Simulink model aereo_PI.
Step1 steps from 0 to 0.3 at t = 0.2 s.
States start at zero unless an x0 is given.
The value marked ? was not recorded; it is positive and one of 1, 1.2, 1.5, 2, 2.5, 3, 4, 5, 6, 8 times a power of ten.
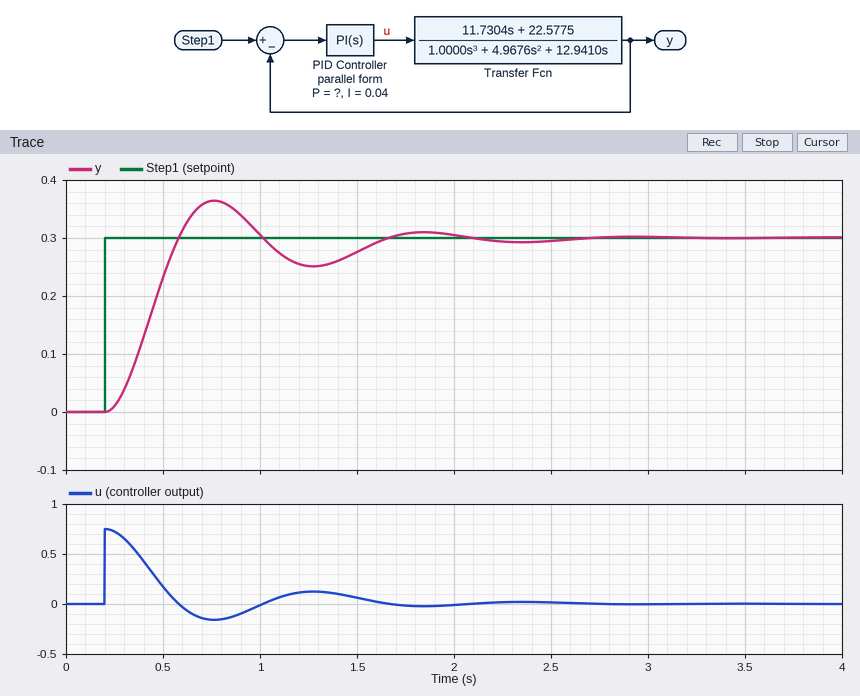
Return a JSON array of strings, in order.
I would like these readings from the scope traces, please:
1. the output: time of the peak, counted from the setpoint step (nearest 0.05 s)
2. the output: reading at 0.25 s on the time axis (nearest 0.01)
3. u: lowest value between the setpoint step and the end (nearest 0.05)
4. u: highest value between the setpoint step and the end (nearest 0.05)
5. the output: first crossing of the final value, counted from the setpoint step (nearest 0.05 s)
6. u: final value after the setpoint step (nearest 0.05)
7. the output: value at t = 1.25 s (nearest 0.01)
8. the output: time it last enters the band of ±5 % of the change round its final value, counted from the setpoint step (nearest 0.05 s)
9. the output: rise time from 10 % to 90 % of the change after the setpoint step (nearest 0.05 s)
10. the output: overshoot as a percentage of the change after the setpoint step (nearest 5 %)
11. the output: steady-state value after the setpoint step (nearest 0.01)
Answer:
["0.55 s", "0.01", "-0.15", "0.75", "0.40 s", "0.00", "0.25", "1.35 s", "0.25 s", "20 %", "0.30"]
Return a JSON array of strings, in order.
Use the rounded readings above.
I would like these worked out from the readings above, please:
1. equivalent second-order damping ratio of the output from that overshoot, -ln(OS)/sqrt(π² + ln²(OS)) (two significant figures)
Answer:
["0.46"]
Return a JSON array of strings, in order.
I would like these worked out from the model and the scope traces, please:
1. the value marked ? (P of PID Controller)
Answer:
["2.5"]
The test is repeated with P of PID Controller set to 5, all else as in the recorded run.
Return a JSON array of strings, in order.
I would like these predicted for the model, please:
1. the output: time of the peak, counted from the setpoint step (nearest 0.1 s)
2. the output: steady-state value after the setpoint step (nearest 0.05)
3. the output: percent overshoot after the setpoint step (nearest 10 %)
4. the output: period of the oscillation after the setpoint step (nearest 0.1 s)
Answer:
["0.4 s", "0.30", "40 %", "0.8 s"]
